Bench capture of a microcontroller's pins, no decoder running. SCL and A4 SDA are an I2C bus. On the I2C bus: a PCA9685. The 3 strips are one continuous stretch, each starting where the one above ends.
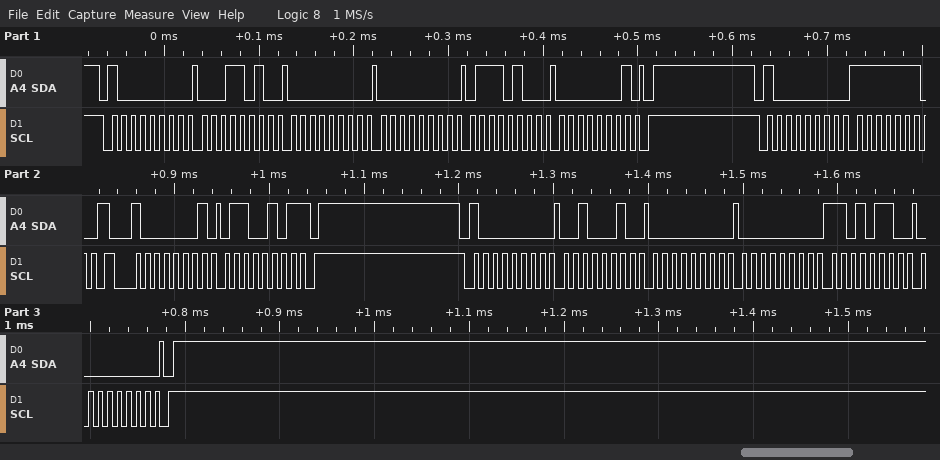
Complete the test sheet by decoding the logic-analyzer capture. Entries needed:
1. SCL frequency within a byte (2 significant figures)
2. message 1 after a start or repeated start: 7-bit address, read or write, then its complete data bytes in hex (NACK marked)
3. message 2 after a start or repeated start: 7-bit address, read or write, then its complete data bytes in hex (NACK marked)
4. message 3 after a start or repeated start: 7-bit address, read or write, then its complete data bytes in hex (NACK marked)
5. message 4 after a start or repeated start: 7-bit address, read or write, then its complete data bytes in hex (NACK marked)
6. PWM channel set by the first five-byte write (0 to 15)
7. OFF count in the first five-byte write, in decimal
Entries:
100 kHz
0x40 write: 1A 00 00 74 01
0x40 write: FE
0x40 read: 65 NACK
0x40 write: 22 00 00 D6 00
5
372
